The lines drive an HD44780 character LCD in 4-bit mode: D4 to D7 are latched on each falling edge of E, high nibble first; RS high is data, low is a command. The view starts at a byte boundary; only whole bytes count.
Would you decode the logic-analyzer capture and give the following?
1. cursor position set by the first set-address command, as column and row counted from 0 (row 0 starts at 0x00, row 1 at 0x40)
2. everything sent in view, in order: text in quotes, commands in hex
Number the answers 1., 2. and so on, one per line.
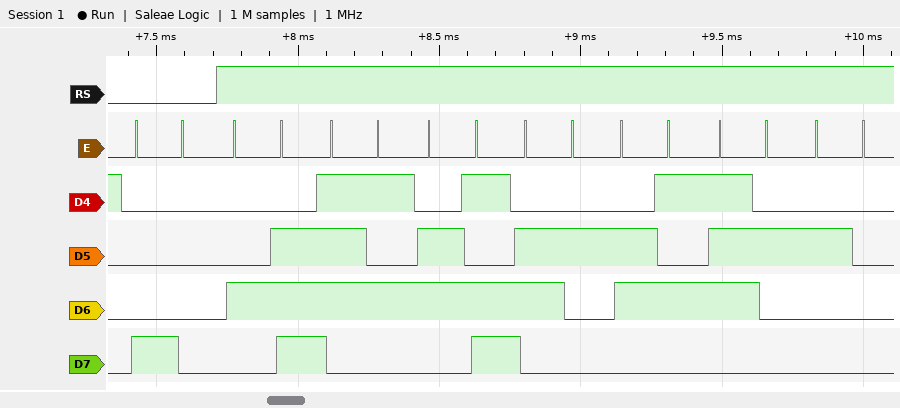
1. column 0, row 0
2. 0x80 "Number "
